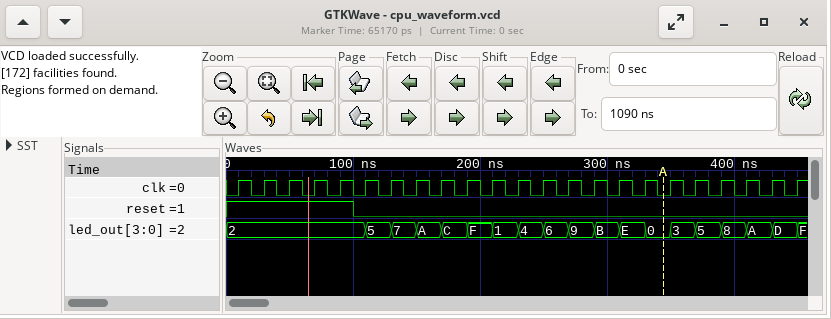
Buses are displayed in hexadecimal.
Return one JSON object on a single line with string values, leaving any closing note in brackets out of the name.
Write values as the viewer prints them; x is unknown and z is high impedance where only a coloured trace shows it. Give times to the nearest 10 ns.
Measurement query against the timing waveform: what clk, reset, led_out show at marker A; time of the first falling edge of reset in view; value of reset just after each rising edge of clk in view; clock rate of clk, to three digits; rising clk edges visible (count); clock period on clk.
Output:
{"what clk, reset, led_out show at marker A": "clk=0, reset=0, led_out=0", "time of the first falling edge of reset in view": "100 ns", "value of reset just after each rising edge of clk in view": "1 1 1 1 1 0 0 0 0 0 0 0 0 0 0 0 0 0 0 0 0 0 0", "clock rate of clk, to three digits": "50.0 MHz", "rising clk edges visible": "23", "clock period on clk": "20 ns"}
